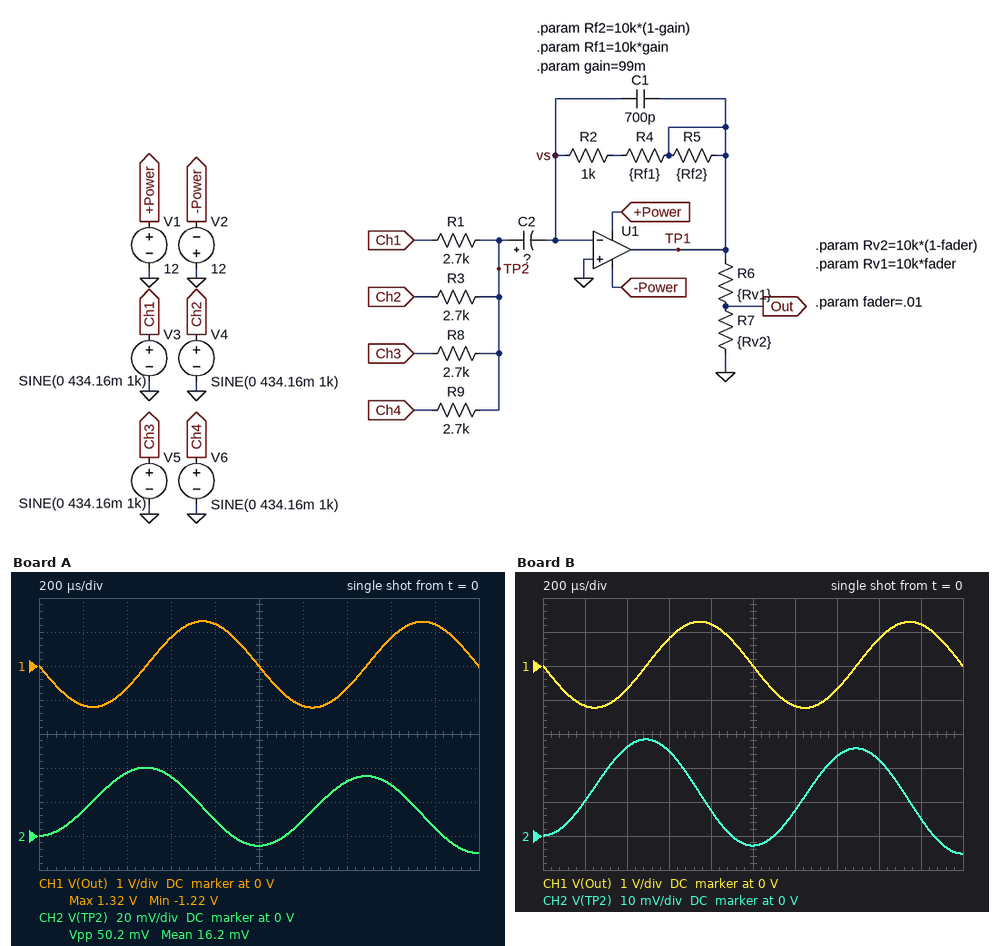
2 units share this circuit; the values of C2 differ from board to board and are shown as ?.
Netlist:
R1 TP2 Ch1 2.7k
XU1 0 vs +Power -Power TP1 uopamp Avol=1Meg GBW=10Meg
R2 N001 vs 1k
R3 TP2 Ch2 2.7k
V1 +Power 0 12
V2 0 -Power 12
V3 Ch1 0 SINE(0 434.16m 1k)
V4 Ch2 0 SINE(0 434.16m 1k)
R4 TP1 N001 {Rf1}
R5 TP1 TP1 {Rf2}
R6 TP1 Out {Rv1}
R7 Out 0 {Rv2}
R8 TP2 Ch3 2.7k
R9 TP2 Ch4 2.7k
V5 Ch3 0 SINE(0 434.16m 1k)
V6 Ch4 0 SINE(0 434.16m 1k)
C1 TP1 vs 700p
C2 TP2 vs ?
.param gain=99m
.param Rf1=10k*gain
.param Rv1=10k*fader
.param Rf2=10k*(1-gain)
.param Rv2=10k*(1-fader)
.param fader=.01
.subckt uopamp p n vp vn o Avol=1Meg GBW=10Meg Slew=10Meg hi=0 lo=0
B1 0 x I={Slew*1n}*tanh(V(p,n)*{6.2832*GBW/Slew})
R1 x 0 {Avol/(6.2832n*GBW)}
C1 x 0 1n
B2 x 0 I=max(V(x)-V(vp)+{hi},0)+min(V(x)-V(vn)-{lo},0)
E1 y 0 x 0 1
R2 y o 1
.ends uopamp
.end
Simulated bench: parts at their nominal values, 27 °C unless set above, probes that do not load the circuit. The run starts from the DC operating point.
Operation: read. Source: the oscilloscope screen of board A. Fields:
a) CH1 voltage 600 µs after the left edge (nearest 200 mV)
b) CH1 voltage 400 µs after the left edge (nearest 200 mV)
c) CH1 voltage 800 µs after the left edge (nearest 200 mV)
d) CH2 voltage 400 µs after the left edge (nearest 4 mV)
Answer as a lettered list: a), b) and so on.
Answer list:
a) 800 mV
b) -600 mV
c) 1.2 V
d) 36 mV
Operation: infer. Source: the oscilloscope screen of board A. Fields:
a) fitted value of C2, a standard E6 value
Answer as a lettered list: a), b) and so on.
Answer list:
a) 4.7 µF
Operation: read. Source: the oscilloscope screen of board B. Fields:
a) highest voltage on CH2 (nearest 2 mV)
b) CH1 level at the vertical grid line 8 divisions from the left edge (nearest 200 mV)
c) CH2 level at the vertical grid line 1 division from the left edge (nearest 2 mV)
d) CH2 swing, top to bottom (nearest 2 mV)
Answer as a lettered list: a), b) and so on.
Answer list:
a) 28 mV
b) 800 mV
c) 10 mV
d) 34 mV
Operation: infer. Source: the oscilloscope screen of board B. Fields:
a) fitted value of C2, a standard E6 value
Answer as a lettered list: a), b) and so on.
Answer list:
a) 6.8 µF
